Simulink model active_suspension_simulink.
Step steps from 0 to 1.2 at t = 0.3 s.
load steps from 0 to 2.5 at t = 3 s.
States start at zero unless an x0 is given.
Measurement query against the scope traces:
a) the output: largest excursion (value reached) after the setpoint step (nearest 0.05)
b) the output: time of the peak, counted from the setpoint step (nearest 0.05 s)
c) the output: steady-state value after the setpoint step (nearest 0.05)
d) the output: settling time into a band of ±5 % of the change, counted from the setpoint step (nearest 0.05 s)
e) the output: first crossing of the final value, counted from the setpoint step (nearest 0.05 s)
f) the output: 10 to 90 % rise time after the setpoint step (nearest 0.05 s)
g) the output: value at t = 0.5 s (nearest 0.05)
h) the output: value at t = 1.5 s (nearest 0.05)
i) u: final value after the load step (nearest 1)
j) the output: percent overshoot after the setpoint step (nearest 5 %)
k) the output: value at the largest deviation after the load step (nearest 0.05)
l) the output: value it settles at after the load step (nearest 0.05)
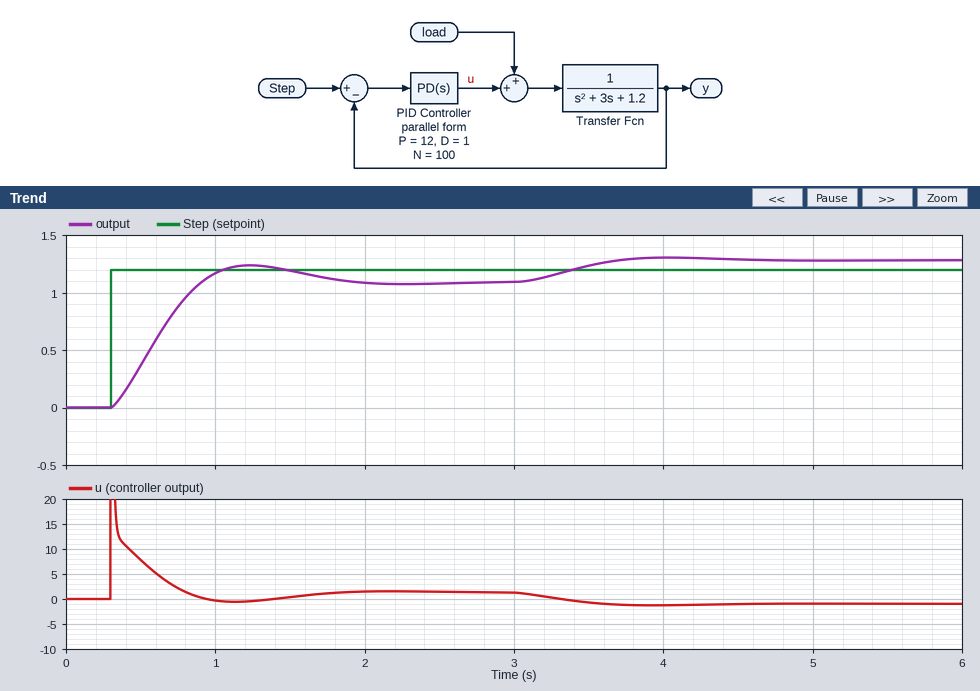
1.25
0.95 s
1.10
1.35 s
0.60 s
0.45 s
0.35
1.20
-1
15 %
1.30
1.30
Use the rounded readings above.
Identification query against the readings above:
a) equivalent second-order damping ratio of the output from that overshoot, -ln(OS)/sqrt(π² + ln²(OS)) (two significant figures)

0.52
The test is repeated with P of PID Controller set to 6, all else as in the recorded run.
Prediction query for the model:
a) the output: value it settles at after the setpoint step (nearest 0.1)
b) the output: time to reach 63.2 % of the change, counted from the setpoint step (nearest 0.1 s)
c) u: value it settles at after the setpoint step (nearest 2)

1.0
0.5 s
2
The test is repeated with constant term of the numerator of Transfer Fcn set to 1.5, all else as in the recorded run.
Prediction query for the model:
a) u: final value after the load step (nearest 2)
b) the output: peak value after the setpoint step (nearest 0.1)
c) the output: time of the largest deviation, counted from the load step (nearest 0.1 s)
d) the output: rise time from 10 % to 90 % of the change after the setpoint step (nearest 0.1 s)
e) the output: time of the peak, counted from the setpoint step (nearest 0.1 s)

-2
1.3
0.8 s
0.3 s
0.7 s
